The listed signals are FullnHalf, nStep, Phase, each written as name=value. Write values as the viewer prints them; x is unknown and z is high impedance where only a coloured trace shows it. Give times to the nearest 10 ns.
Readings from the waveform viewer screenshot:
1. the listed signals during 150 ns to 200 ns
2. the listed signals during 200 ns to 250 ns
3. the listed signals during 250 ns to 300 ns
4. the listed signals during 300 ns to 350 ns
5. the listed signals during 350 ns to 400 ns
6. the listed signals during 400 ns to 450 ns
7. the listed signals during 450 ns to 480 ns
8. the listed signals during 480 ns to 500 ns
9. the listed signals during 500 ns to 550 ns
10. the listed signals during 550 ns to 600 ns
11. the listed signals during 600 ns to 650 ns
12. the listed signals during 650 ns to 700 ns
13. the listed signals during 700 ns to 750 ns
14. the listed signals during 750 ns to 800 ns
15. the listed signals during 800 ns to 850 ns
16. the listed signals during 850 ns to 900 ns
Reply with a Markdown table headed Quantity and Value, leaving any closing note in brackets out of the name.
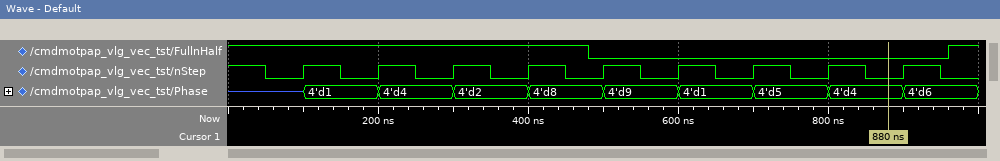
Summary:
| Quantity | Value |
|---|---|
| the listed signals during 150 ns to 200 ns | FullnHalf=1, nStep=0, Phase=4'd1 |
| the listed signals during 200 ns to 250 ns | FullnHalf=1, nStep=1, Phase=4'd4 |
| the listed signals during 250 ns to 300 ns | FullnHalf=1, nStep=0, Phase=4'd4 |
| the listed signals during 300 ns to 350 ns | FullnHalf=1, nStep=1, Phase=4'd2 |
| the listed signals during 350 ns to 400 ns | FullnHalf=1, nStep=0, Phase=4'd2 |
| the listed signals during 400 ns to 450 ns | FullnHalf=1, nStep=1, Phase=4'd8 |
| the listed signals during 450 ns to 480 ns | FullnHalf=1, nStep=0, Phase=4'd8 |
| the listed signals during 480 ns to 500 ns | FullnHalf=0, nStep=0, Phase=4'd8 |
| the listed signals during 500 ns to 550 ns | FullnHalf=0, nStep=1, Phase=4'd9 |
| the listed signals during 550 ns to 600 ns | FullnHalf=0, nStep=0, Phase=4'd9 |
| the listed signals during 600 ns to 650 ns | FullnHalf=0, nStep=1, Phase=4'd1 |
| the listed signals during 650 ns to 700 ns | FullnHalf=0, nStep=0, Phase=4'd1 |
| the listed signals during 700 ns to 750 ns | FullnHalf=0, nStep=1, Phase=4'd5 |
| the listed signals during 750 ns to 800 ns | FullnHalf=0, nStep=0, Phase=4'd5 |
| the listed signals during 800 ns to 850 ns | FullnHalf=0, nStep=1, Phase=4'd4 |
| the listed signals during 850 ns to 900 ns | FullnHalf=0, nStep=0, Phase=4'd4 |
